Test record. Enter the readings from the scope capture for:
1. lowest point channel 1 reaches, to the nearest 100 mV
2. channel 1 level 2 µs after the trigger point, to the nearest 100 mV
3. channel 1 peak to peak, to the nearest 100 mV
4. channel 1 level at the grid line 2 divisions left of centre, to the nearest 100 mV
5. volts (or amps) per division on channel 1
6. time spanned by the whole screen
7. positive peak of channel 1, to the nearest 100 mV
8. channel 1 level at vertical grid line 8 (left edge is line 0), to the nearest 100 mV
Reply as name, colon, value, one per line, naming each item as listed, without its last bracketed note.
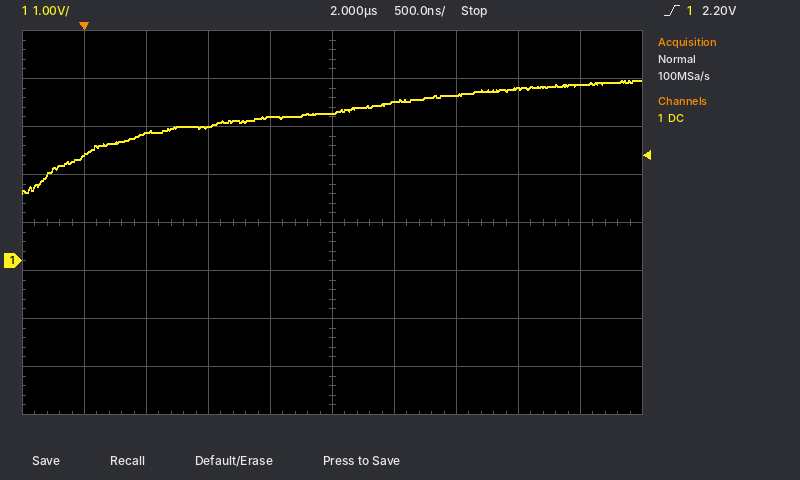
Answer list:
lowest point channel 1 reaches, to the nearest 100 mV: 1.4 V
channel 1 level 2 µs after the trigger point, to the nearest 100 mV: 3.1 V
channel 1 peak to peak, to the nearest 100 mV: 2.4 V
channel 1 level at the grid line 2 divisions left of centre, to the nearest 100 mV: 2.8 V
volts (or amps) per division on channel 1: 1 V
time spanned by the whole screen: 5 µs
positive peak of channel 1, to the nearest 100 mV: 3.8 V
channel 1 level at vertical grid line 8 (left edge is line 0), to the nearest 100 mV: 3.6 V
